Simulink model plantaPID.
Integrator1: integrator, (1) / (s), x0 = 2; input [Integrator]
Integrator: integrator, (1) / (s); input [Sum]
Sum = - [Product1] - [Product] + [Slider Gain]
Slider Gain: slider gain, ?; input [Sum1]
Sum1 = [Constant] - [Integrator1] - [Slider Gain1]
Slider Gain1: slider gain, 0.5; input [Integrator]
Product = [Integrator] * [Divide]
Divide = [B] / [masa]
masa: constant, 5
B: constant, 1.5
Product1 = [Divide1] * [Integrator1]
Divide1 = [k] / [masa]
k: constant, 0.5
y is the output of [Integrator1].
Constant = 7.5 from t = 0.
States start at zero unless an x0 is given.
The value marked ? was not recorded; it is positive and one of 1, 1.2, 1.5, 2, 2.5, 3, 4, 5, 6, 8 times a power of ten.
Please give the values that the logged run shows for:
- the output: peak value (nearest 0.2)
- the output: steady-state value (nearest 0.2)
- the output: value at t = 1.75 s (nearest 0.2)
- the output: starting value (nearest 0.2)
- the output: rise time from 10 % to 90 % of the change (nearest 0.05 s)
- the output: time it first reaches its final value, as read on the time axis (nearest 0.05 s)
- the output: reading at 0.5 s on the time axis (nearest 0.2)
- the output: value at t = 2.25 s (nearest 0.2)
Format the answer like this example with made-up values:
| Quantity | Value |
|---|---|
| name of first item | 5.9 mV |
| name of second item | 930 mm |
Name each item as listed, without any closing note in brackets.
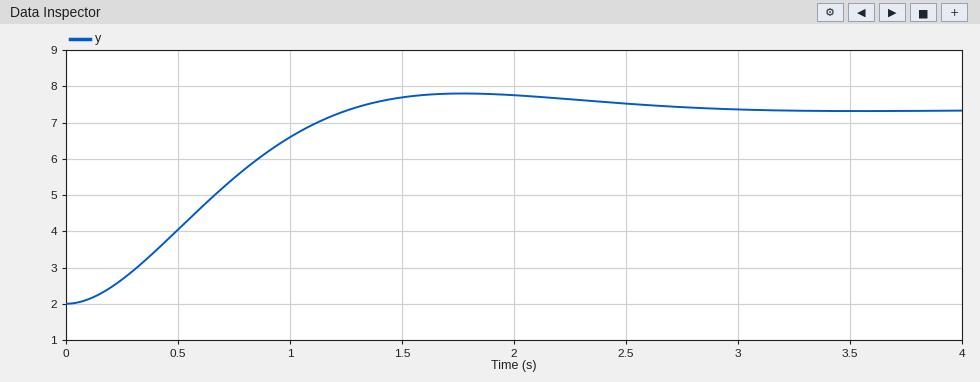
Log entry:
| Quantity | Value |
|---|---|
| the output: peak value | 7.8 |
| the output: steady-state value | 7.4 |
| the output: value at t = 1.75 s | 7.8 |
| the output: starting value | 2.0 |
| the output: rise time from 10 % to 90 % of the change | 0.85 s |
| the output: time it first reaches its final value, as read on the time axis | 1.25 s |
| the output: reading at 0.5 s on the time axis | 4.0 |
| the output: value at t = 2.25 s | 7.6 |
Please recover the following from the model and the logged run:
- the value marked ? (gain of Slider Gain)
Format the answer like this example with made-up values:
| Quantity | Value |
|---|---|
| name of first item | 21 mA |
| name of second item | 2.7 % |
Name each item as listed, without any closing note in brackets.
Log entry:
| Quantity | Value |
|---|---|
| the value marked ? | 5 |
